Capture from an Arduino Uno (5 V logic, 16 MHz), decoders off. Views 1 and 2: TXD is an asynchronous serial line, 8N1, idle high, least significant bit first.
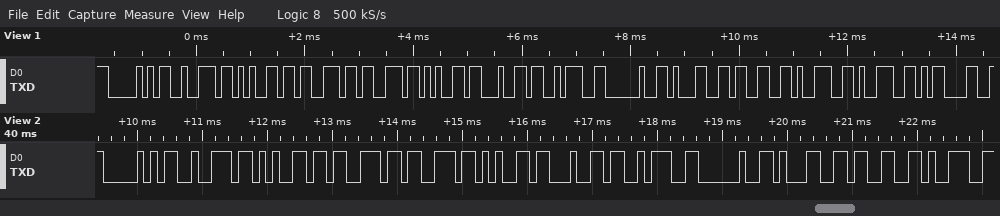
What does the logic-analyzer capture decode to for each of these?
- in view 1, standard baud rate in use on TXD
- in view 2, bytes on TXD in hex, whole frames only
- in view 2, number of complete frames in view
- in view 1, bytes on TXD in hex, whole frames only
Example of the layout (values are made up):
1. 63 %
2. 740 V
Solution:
1. 9600 baud
2. 0x50 0x72 0x65 0x73 0x73 0x65 0x64 0x3A 0x20 0x31 0x33 0x39
3. 12
4. 0x50 0x72 0x65 0x73 0x73 0x65 0x64 0x3A 0x20 0x31 0x33 0x39 0x39 0x0D
